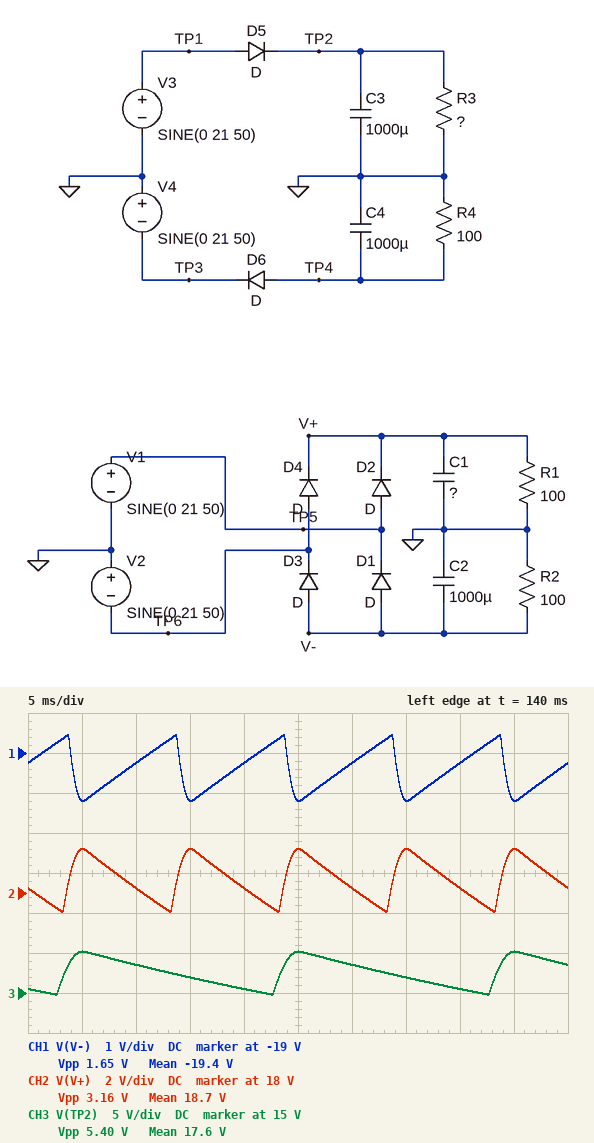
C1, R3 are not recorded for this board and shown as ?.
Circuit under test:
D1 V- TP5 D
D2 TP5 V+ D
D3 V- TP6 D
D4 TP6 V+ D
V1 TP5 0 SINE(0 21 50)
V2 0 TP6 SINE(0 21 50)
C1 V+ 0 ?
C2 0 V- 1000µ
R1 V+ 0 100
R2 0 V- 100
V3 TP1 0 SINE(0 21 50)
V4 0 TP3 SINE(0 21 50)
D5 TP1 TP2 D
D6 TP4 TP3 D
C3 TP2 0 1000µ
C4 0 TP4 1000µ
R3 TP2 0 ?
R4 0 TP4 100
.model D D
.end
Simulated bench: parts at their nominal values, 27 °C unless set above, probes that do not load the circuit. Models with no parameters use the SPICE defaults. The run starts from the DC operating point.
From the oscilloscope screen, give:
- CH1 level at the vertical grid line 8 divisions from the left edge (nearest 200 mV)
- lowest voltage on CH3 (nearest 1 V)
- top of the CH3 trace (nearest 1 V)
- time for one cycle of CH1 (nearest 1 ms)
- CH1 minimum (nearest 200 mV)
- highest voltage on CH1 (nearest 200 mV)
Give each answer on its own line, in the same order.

-19.2 V
15 V
20 V
10 ms
-20.2 V
-18.6 V
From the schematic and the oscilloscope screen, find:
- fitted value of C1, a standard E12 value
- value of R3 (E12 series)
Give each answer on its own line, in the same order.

470 µF
56 Ω
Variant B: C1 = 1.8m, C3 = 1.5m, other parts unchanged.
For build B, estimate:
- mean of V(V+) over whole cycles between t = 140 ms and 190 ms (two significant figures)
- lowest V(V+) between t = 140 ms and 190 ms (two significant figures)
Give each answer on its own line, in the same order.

20 V
19 V
